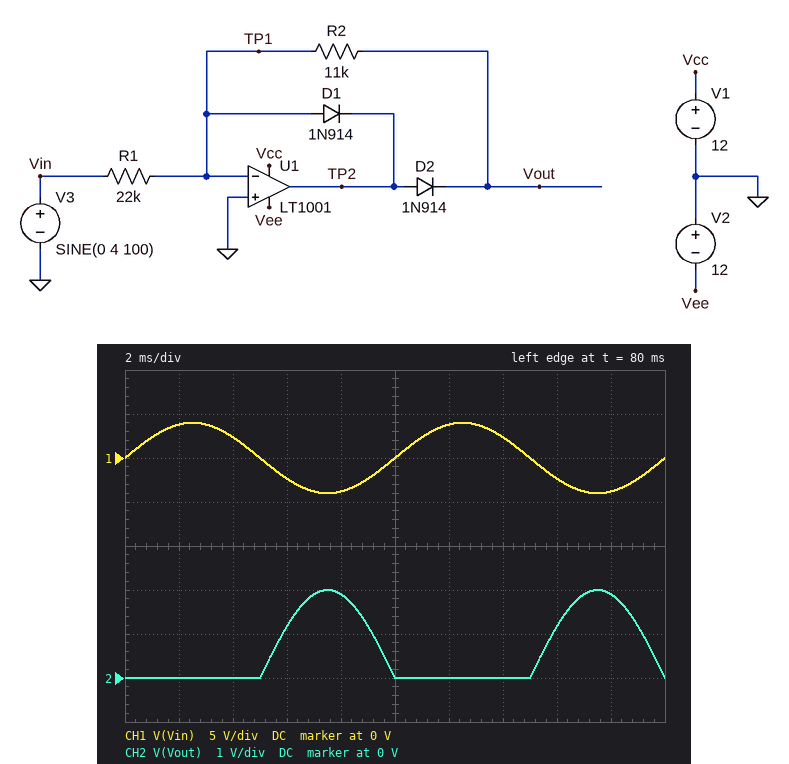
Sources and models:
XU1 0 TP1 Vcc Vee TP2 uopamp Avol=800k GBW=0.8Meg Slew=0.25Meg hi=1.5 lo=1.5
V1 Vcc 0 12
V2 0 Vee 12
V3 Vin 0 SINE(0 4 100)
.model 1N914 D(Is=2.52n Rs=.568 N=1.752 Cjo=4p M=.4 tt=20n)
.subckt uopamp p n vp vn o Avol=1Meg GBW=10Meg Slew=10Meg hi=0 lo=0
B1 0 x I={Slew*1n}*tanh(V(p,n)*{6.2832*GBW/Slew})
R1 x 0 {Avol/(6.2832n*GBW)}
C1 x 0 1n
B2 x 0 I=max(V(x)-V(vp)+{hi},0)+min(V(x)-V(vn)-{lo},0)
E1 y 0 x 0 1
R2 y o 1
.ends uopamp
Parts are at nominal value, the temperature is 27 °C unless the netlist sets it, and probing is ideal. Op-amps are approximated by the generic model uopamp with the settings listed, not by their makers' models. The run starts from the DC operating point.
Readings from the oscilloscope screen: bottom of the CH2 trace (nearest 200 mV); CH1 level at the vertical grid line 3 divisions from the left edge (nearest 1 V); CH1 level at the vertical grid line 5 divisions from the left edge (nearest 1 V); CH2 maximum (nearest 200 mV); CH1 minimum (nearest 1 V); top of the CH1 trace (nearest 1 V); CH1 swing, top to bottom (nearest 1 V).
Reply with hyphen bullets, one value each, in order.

- 0 V
- -2 V
- 0 V
- 2.0 V
- -4 V
- 4 V
- 8 V
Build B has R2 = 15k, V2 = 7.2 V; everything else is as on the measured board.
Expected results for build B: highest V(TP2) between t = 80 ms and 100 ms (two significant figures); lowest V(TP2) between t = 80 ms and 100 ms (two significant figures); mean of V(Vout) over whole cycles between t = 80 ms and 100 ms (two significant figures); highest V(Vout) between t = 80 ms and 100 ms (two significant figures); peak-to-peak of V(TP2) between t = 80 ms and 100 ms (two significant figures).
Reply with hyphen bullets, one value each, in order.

- 3.2 V
- -510 mV
- 870 mV
- 2.7 V
- 3.7 V
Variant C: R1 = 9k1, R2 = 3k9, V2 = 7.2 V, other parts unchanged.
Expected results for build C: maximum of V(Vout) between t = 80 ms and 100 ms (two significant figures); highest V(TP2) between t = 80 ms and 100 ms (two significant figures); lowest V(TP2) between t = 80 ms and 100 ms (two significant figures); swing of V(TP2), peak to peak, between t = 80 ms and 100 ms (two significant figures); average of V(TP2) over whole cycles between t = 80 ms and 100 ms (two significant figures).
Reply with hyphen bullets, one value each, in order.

- 1.7 V
- 2.3 V
- -550 mV
- 2.8 V
- 550 mV
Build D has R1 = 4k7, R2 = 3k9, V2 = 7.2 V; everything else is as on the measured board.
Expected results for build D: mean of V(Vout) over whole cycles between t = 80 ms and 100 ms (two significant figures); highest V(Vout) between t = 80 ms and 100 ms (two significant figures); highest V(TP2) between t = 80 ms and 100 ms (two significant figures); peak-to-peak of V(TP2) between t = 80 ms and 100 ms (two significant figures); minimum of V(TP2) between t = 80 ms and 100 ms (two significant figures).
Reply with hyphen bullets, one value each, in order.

- 1.1 V
- 3.3 V
- 3.9 V
- 4.5 V
- -580 mV
